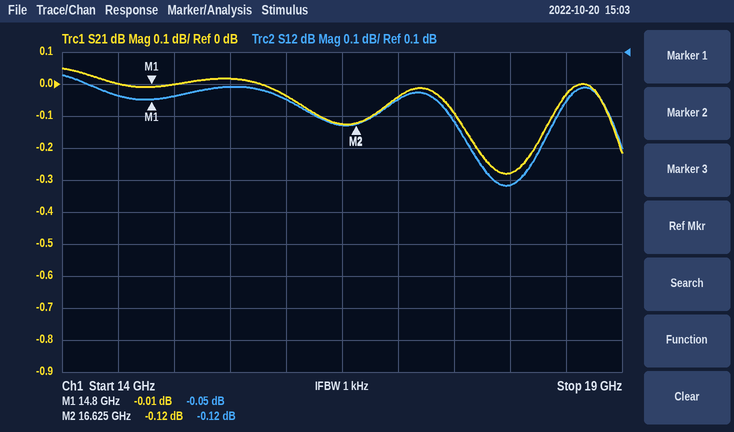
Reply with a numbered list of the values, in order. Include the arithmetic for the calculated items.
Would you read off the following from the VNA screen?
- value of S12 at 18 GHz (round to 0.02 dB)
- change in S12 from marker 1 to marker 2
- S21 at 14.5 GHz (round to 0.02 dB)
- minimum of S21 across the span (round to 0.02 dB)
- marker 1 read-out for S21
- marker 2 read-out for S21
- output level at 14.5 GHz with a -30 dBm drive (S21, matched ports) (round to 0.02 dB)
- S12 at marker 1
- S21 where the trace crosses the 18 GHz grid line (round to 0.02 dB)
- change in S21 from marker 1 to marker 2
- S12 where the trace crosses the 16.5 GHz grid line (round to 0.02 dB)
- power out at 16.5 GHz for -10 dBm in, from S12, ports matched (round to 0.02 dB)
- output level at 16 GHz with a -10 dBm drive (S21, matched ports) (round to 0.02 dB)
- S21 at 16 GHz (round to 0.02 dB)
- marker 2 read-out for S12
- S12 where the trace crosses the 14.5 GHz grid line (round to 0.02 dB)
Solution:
1. -0.32 dB
2. -0.12 − (-0.05) = -0.07 dB
3. 0.00 dB
4. -0.28 dB
5. -0.01 dB
6. -0.12 dB
7. -30 dBm + (0.00 dB) = -30.00 dBm
8. -0.05 dB
9. -0.28 dB
10. -0.12 − (-0.01) = -0.11 dB
11. -0.12 dB
12. -10 dBm + (-0.12 dB) = -10.12 dBm
13. -10 dBm + (-0.04 dB) = -10.04 dBm
14. -0.04 dB
15. -0.12 dB
16. -0.04 dB
